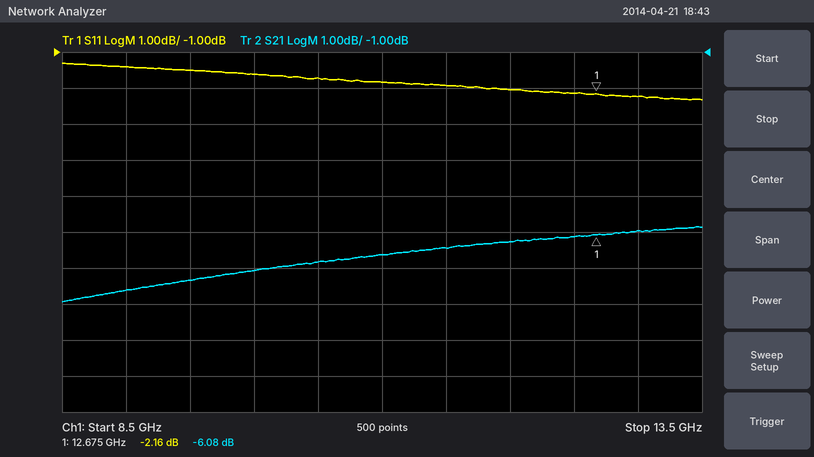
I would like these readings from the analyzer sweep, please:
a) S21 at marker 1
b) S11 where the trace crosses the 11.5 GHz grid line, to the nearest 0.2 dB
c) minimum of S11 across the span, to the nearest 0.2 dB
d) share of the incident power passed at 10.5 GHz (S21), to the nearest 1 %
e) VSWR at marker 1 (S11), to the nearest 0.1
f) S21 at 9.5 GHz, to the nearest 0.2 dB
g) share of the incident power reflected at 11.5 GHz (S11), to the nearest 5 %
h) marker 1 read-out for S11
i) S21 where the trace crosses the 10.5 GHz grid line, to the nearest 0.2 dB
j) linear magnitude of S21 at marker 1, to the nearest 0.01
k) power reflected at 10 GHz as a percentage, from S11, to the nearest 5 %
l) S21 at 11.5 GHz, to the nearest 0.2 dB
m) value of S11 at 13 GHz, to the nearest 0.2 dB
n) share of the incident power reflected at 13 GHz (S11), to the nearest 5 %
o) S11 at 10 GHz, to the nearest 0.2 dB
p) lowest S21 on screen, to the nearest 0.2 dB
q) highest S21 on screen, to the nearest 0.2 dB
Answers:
-6.08 dB
-2.0 dB
-2.4 dB
21 %
8.1
-7.4 dB
65 %
-2.16 dB
-6.8 dB
0.50
70 %
-6.4 dB
-2.2 dB
60 %
-1.6 dB
-8.0 dB
-5.8 dB
